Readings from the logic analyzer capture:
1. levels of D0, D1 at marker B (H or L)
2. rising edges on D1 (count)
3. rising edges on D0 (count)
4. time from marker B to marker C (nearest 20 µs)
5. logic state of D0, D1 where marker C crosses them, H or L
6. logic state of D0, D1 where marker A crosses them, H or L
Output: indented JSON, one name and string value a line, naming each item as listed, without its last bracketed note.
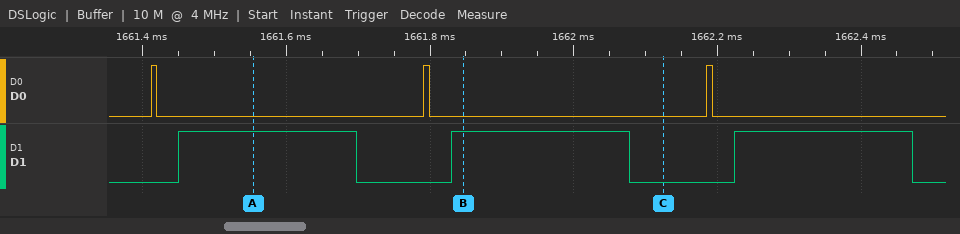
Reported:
{
  "levels of D0, D1 at marker B": "D0=L, D1=H",
  "rising edges on D1": "3",
  "rising edges on D0": "3",
  "time from marker B to marker C": "280 µs",
  "logic state of D0, D1 where marker C crosses them, H or L": "D0=L, D1=L",
  "logic state of D0, D1 where marker A crosses them, H or L": "D0=L, D1=H"
}
